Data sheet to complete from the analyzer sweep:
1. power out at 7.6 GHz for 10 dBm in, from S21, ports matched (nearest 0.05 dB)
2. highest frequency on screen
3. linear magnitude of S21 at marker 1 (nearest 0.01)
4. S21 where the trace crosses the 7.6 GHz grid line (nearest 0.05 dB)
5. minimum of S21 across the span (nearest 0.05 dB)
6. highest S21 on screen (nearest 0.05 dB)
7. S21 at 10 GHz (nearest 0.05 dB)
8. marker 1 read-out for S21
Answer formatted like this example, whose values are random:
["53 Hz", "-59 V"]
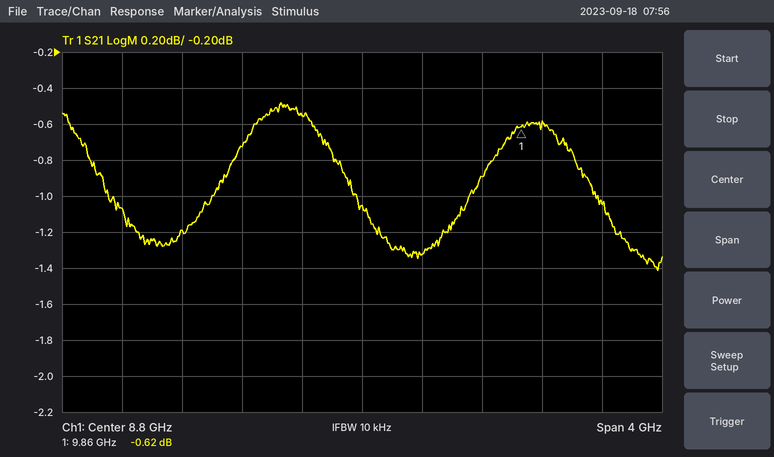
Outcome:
["8.80 dBm", "10.8 GHz", "0.93", "-1.20 dB", "-1.40 dB", "-0.50 dB", "-0.60 dB", "-0.62 dB"]
